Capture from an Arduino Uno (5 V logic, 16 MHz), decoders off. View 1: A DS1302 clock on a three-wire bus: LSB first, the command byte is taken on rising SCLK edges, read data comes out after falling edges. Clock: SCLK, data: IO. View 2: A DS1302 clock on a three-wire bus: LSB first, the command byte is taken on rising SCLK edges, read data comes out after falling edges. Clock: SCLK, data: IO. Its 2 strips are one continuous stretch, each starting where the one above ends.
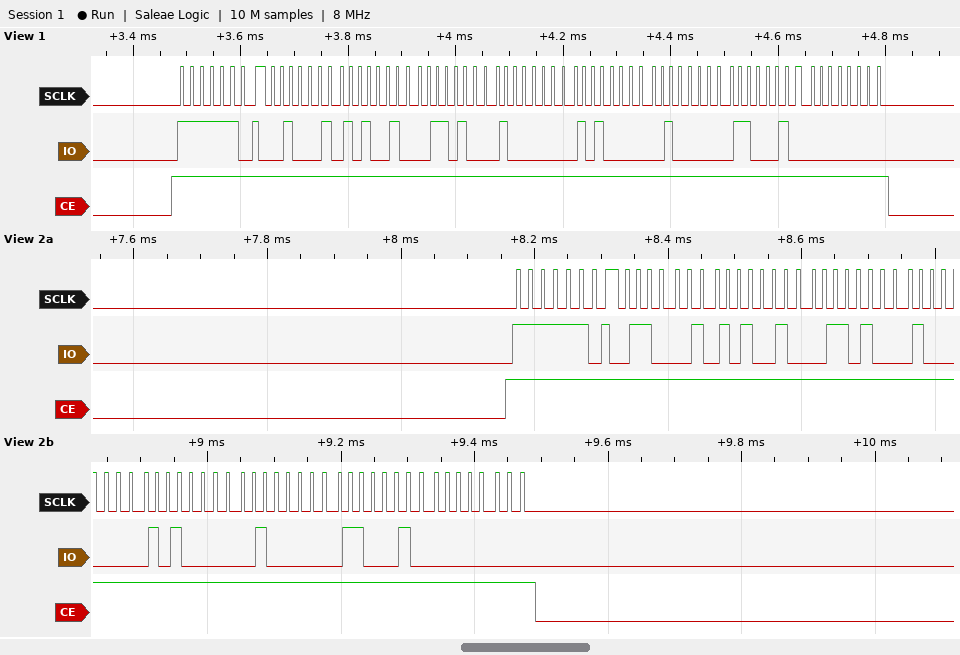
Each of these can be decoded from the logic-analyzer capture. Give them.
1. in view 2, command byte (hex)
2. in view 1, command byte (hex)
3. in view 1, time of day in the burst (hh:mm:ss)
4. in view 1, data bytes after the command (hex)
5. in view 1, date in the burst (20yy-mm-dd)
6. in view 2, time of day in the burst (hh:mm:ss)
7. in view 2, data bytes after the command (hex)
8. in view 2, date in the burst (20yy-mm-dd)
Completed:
0xBF
0xBF
16:25:44
44 25 16 01 05 02 23 00
2023-05-01
16:25:46
46 25 16 01 05 02 23 00
2023-05-01
